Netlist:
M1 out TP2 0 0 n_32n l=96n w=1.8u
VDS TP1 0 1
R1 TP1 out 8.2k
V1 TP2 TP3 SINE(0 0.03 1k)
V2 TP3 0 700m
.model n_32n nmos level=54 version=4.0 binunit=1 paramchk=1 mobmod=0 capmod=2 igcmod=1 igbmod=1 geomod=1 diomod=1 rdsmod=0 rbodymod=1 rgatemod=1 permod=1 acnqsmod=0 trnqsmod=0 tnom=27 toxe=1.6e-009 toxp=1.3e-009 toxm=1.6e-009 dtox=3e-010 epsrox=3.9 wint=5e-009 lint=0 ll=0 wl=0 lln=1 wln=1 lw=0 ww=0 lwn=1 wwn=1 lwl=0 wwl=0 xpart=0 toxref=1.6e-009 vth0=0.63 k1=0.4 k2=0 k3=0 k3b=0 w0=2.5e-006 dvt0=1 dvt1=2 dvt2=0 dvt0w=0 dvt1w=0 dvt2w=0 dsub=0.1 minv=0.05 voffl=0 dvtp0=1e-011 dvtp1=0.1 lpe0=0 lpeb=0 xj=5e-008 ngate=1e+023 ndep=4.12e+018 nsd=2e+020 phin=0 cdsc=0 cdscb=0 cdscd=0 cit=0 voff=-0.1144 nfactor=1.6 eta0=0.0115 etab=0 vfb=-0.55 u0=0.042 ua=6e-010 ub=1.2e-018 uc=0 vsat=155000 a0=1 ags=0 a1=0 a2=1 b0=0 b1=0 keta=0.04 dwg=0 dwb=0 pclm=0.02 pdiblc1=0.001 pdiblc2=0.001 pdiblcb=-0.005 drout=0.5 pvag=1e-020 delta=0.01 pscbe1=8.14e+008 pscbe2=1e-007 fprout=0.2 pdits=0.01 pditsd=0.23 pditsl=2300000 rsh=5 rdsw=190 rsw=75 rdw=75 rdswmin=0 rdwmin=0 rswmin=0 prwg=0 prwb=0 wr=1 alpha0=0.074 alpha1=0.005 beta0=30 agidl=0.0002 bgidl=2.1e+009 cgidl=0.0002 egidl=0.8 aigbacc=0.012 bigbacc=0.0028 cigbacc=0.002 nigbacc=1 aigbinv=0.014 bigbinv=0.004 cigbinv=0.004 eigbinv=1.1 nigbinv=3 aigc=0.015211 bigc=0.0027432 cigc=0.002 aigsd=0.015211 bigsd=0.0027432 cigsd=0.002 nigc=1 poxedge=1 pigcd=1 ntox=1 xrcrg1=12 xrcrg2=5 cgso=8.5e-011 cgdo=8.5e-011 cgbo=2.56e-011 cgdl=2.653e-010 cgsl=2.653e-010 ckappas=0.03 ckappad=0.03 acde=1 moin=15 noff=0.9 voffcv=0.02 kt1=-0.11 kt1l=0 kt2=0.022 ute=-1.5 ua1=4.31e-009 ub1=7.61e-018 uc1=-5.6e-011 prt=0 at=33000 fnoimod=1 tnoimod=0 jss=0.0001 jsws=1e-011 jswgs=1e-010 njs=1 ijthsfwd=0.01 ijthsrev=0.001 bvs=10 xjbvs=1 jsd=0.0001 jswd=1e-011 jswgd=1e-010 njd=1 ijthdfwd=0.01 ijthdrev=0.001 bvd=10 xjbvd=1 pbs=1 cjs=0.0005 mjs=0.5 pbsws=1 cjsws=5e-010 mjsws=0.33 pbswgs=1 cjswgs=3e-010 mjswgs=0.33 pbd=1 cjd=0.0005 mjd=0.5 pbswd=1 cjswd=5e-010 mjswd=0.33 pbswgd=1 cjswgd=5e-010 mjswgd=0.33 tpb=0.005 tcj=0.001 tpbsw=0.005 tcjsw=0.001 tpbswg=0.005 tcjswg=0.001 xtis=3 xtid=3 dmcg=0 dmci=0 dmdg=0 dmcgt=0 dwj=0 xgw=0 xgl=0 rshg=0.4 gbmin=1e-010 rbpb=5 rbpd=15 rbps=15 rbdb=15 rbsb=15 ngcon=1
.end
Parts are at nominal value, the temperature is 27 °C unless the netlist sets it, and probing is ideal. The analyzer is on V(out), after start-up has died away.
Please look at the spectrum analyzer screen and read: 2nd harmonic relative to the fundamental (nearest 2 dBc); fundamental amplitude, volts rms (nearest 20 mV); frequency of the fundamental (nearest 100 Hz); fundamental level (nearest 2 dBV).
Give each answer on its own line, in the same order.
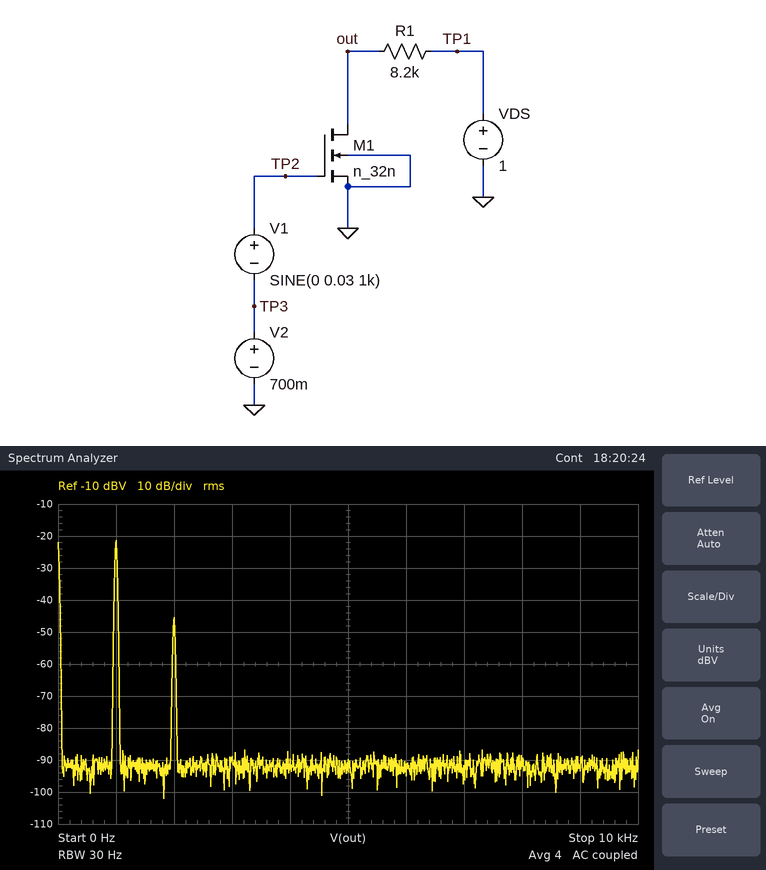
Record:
-24 dBc
80 mV
1.0 kHz
-22 dBV
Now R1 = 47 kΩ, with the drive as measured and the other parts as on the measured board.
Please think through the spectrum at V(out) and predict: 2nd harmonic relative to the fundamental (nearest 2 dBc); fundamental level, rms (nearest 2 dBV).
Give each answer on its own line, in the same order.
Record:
-10 dBc
-34 dBV
